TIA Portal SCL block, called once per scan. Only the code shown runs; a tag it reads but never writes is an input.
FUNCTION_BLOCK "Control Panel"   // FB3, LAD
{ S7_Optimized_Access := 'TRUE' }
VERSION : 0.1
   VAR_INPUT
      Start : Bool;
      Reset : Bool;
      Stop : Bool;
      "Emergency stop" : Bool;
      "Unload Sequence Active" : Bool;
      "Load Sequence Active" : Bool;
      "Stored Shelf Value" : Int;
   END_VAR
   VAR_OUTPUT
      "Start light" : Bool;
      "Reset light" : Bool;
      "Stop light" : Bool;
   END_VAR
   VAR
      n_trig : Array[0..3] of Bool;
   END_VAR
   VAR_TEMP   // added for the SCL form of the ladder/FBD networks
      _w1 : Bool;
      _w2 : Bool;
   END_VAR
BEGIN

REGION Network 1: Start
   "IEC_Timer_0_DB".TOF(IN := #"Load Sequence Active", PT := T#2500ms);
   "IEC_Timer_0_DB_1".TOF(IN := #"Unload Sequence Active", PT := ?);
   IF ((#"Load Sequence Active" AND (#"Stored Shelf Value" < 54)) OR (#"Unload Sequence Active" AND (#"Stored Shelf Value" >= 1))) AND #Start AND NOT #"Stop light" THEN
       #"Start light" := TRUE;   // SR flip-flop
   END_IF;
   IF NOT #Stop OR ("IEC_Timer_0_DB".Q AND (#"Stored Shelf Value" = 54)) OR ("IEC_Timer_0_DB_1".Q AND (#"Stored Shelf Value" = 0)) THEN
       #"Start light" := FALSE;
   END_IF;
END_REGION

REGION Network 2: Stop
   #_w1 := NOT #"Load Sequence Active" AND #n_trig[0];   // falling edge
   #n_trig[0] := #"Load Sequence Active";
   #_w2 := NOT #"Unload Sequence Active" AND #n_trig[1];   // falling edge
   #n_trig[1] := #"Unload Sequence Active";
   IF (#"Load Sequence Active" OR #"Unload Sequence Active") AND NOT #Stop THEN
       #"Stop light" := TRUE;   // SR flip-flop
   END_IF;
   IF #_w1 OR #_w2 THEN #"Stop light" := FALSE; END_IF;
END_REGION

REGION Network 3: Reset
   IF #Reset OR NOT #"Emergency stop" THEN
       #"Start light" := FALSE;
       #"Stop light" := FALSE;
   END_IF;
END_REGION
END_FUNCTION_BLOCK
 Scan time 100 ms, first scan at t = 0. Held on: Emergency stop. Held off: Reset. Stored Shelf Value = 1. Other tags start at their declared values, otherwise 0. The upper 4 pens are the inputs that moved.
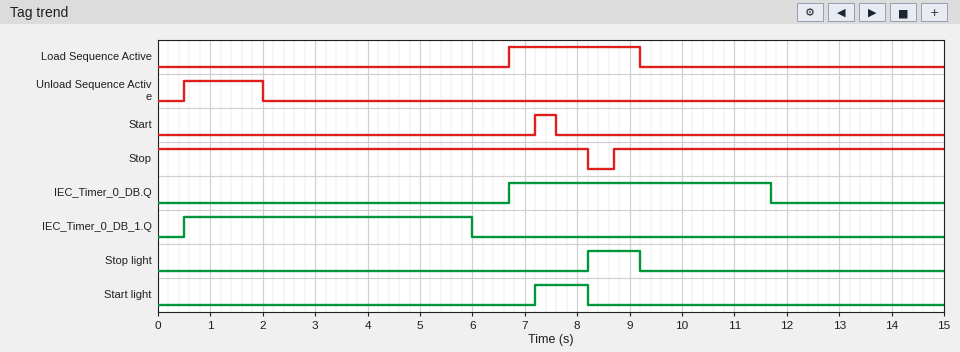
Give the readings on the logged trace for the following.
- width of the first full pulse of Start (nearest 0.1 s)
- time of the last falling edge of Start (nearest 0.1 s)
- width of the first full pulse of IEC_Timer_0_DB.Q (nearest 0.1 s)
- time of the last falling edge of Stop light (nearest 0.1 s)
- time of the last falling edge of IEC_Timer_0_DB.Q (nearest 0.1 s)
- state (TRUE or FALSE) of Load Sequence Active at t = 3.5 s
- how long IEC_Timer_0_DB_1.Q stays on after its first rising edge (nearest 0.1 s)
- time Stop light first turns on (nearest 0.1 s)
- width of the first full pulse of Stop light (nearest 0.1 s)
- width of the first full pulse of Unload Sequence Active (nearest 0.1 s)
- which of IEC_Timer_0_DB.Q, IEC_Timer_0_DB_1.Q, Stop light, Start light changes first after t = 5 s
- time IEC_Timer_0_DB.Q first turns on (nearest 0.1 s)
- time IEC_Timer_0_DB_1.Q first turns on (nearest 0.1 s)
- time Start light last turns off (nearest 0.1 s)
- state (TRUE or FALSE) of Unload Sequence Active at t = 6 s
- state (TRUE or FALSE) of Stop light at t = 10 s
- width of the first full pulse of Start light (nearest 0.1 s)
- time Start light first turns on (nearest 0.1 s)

0.4 s
7.6 s
5.0 s
9.2 s
11.7 s
FALSE
5.5 s
8.2 s
1.0 s
1.5 s
IEC_Timer_0_DB_1.Q
6.7 s
0.5 s
8.2 s
FALSE
FALSE
1.0 s
7.2 s
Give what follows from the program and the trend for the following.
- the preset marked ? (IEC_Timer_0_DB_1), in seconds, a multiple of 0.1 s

4.0 s
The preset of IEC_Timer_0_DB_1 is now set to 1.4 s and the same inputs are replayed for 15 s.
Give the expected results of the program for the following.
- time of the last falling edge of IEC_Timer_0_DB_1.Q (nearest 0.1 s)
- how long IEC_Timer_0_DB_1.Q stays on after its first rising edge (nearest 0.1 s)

3.4 s
2.9 s
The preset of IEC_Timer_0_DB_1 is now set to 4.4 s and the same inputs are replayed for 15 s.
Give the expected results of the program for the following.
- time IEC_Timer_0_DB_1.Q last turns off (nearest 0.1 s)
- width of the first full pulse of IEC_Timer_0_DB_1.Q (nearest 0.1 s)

6.4 s
5.9 s
